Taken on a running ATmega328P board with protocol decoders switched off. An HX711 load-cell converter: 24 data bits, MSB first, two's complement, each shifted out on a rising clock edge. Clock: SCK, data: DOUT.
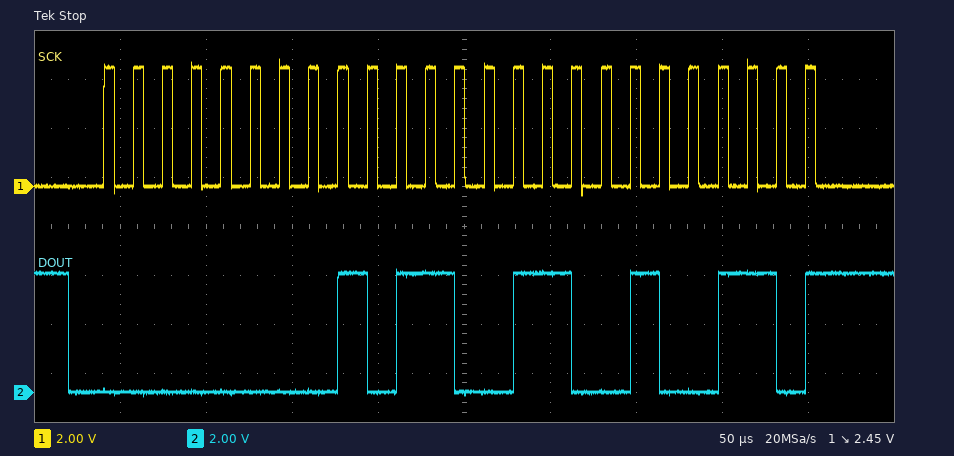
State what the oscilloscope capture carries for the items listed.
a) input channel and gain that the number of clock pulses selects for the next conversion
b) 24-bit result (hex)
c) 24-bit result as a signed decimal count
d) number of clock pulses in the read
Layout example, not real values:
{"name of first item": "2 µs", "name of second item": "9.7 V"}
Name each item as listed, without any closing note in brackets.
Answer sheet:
{"input channel and gain that the number of clock pulses selects for the next conversion": "channel A, gain 128", "24-bit result": "0x00B326", "24-bit result as a signed decimal count": "45862", "number of clock pulses in the read": "25"}
